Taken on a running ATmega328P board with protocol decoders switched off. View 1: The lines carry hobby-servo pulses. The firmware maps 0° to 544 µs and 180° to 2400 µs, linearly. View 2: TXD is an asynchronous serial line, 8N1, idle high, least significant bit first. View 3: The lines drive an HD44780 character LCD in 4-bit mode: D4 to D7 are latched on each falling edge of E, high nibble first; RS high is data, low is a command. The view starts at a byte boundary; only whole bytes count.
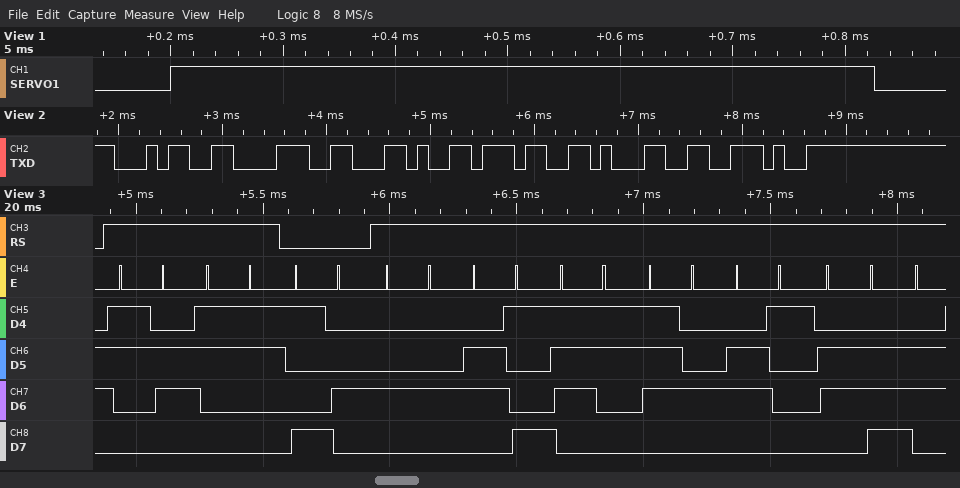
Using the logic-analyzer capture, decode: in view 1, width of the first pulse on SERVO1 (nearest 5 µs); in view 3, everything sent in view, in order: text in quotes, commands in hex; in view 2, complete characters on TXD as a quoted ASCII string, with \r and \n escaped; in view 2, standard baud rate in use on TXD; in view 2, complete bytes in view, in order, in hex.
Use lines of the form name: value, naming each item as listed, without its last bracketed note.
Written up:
in view 1, width of the first pulse on SERVO1: 625 µs
in view 3, everything sent in view, in order: text in quotes, commands in hex: "63" 0x94 "Distan"
in view 2, complete characters on TXD as a quoted ASCII string, with \r and \n escaped: "48,71."
in view 2, standard baud rate in use on TXD: 9600 baud
in view 2, complete bytes in view, in order, in hex: 34 38 2C 37 31 2E
